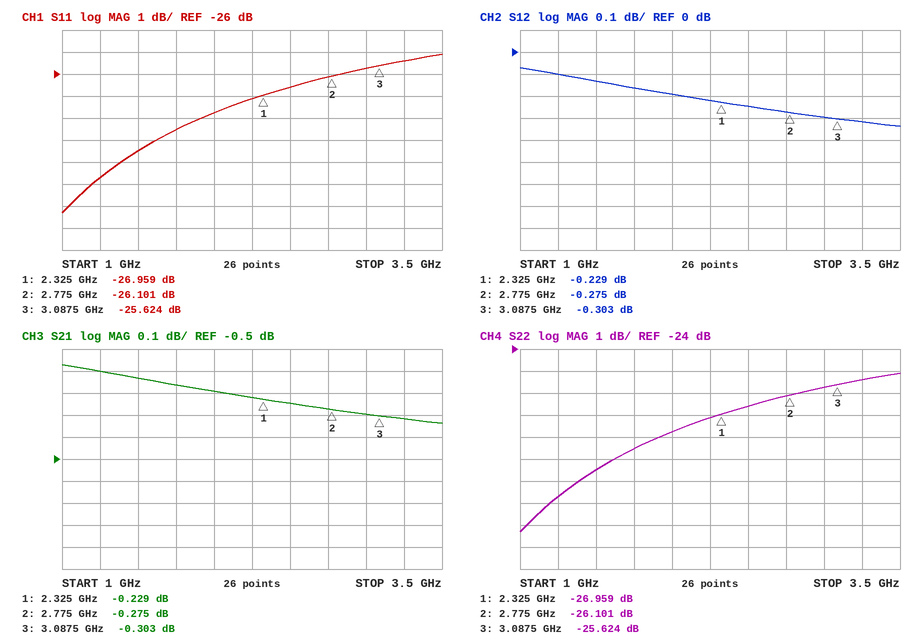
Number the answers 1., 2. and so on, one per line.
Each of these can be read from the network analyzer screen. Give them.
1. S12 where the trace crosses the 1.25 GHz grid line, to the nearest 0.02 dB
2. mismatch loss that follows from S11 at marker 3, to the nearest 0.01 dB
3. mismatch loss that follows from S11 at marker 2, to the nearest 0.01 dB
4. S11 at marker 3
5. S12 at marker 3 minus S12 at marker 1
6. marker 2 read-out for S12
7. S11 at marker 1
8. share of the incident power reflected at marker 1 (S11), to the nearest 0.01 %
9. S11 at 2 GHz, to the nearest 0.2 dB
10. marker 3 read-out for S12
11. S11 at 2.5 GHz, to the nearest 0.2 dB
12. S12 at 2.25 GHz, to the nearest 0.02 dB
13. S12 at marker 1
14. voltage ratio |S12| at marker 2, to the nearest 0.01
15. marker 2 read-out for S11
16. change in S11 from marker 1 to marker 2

1. -0.10 dB
2. 0.01 dB
3. 0.01 dB
4. -25.624 dB
5. -0.074 dB
6. -0.275 dB
7. -26.959 dB
8. 0.20 %
9. -27.8 dB
10. -0.303 dB
11. -26.6 dB
12. -0.22 dB
13. -0.229 dB
14. 0.97
15. -26.101 dB
16. 0.858 dB
